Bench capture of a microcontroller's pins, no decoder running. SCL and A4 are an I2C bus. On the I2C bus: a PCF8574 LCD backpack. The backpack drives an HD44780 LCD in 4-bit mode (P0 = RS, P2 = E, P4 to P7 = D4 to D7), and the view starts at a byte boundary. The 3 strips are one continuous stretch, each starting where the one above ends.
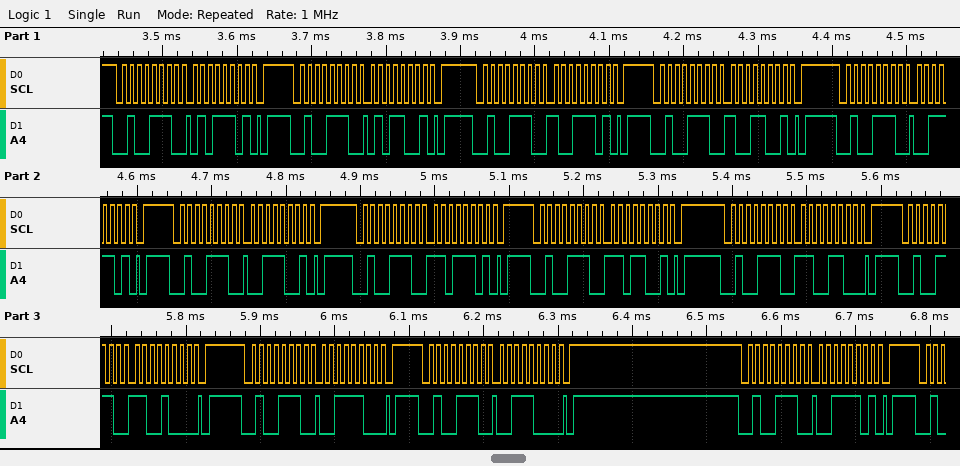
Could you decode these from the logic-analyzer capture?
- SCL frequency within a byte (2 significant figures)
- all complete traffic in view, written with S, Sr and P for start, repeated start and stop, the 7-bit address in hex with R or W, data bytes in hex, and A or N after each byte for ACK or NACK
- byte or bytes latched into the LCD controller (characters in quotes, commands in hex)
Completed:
100 kHz
S 27W A 5D A P S 27W A 59 A P S 27W A 9D A P S 27W A 99 A P S 27W A 3D A P S 27W A 39 A P S 27W A DD A P S 27W A D9 A P S 27W A CC A P S 27W A C8 A P S 27W A 3C A P S 27W A 38 A P S 27W A 3D A P
'Y' '=' 0xC3
